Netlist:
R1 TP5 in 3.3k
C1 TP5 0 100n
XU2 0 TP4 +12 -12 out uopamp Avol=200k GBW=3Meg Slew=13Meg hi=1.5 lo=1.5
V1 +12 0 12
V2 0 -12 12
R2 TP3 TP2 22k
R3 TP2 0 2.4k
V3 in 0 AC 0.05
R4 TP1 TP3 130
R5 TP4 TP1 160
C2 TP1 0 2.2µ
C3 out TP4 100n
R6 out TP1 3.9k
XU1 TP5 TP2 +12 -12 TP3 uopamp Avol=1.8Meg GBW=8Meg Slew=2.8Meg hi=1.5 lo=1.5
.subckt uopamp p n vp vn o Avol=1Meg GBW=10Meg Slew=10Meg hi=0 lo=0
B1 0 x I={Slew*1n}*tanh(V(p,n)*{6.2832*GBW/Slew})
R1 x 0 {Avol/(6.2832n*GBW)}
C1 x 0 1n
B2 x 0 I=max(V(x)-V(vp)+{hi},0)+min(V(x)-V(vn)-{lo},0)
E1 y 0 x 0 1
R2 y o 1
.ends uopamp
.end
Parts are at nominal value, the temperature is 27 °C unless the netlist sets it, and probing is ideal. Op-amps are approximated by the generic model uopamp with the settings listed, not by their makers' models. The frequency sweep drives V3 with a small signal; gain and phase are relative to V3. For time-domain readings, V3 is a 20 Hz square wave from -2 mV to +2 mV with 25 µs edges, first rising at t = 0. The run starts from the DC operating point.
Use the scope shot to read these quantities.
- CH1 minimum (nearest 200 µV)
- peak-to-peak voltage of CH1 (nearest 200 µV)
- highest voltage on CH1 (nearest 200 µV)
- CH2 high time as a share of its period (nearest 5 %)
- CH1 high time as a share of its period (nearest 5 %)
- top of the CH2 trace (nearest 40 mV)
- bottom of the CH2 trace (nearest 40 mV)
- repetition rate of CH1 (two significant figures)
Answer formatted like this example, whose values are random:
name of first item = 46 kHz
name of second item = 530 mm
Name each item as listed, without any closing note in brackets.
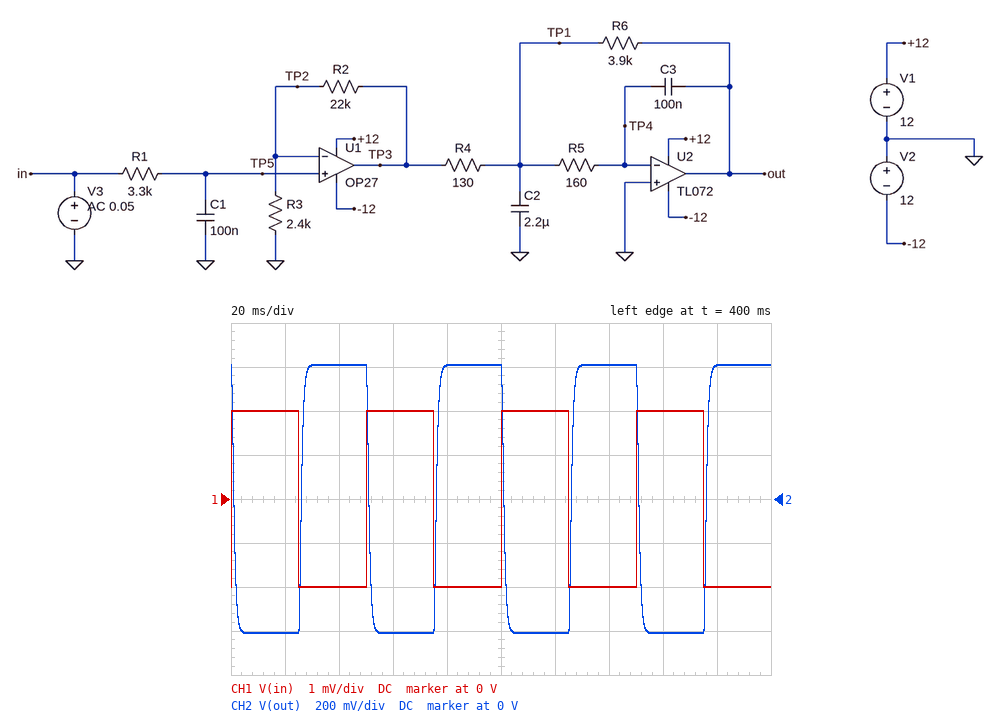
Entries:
CH1 minimum = -2.0 mV
peak-to-peak voltage of CH1 = 4.0 mV
highest voltage on CH1 = 2.0 mV
CH2 high time as a share of its period = 50 %
CH1 high time as a share of its period = 50 %
top of the CH2 trace = 600 mV
bottom of the CH2 trace = -600 mV
repetition rate of CH1 = 20 Hz
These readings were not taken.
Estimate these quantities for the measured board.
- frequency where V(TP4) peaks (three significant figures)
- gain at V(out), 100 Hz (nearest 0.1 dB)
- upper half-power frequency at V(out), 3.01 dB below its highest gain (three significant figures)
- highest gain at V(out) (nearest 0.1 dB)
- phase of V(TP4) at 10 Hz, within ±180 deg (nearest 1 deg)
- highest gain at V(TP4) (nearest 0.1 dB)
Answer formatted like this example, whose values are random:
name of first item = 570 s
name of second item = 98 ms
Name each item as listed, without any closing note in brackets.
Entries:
frequency where V(TP4) peaks = 291 Hz
gain at V(out), 100 Hz = 48.7 dB
upper half-power frequency at V(out), 3.01 dB below its highest gain = 187 Hz
highest gain at V(out) = 49.7 dB
phase of V(TP4) at 10 Hz, within ±180 deg = 29 deg
highest gain at V(TP4) = -36.6 dB
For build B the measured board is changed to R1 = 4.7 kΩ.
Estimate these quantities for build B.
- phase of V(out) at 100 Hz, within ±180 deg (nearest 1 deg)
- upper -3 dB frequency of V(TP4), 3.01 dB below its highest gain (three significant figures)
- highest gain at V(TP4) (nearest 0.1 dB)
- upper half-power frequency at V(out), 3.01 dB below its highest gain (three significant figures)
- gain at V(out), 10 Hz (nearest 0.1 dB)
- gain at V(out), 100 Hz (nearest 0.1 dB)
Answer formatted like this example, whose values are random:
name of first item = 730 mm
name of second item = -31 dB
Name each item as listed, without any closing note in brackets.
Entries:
phase of V(out) at 100 Hz, within ±180 deg = 133 deg
upper -3 dB frequency of V(TP4), 3.01 dB below its highest gain = 548 Hz
highest gain at V(TP4) = -37.5 dB
upper half-power frequency at V(out), 3.01 dB below its highest gain = 169 Hz
gain at V(out), 10 Hz = 49.7 dB
gain at V(out), 100 Hz = 48.5 dB
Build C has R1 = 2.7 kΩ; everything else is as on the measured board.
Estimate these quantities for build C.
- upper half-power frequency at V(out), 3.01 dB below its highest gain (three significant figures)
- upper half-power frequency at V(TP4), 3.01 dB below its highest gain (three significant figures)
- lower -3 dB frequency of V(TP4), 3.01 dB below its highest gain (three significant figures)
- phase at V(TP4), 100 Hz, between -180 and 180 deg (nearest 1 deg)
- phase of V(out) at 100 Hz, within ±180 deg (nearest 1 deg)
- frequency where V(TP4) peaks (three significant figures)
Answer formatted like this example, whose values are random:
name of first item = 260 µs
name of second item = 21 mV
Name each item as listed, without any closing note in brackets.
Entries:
upper half-power frequency at V(out), 3.01 dB below its highest gain = 194 Hz
upper half-power frequency at V(TP4), 3.01 dB below its highest gain = 686 Hz
lower -3 dB frequency of V(TP4), 3.01 dB below its highest gain = 127 Hz
phase at V(TP4), 100 Hz, between -180 and 180 deg = 41 deg
phase of V(out) at 100 Hz, within ±180 deg = 140 deg
frequency where V(TP4) peaks = 312 Hz
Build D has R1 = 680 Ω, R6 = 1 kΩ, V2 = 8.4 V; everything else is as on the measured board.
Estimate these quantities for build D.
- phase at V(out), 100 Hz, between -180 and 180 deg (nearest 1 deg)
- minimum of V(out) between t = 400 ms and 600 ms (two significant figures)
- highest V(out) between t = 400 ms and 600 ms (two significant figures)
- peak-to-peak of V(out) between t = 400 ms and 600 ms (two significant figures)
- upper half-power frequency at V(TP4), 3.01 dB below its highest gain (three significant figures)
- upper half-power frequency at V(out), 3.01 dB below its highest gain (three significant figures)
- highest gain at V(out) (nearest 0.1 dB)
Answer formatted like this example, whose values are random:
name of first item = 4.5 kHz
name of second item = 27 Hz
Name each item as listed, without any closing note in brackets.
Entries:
phase at V(out), 100 Hz, between -180 and 180 deg = 169 deg
minimum of V(out) between t = 400 ms and 600 ms = -180 mV
highest V(out) between t = 400 ms and 600 ms = 180 mV
peak-to-peak of V(out) between t = 400 ms and 600 ms = 360 mV
upper half-power frequency at V(TP4), 3.01 dB below its highest gain = 1.39 kHz
upper half-power frequency at V(out), 3.01 dB below its highest gain = 873 Hz
highest gain at V(out) = 37.9 dB
